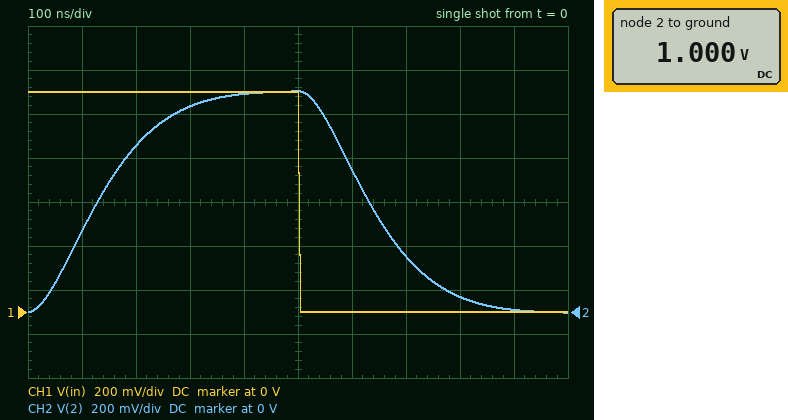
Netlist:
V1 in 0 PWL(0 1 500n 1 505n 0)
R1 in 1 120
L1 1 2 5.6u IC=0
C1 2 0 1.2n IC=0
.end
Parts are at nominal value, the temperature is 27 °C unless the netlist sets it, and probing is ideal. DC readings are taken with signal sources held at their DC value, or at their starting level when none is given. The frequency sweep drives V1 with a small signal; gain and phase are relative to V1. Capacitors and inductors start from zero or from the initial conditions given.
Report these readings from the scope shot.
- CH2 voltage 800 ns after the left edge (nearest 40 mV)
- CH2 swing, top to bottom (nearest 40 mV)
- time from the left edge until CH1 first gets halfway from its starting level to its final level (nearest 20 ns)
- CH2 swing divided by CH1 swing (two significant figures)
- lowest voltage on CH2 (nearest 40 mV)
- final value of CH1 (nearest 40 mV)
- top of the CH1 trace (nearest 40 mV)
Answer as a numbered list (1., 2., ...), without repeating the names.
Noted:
1. 80 mV
2. 1.00 V
3. 500 ns
4. 1.0
5. 0 V
6. 0 V
7. 1.00 V
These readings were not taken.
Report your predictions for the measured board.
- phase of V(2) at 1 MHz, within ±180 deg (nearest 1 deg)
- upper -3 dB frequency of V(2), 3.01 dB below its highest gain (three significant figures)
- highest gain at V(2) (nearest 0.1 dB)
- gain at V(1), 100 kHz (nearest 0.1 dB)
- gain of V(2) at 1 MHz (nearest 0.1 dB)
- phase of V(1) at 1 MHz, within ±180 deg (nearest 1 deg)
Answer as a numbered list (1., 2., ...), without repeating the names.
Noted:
1. -51 deg
2. 1.50 MHz
3. 0 dB
4. 0 dB
5. -1.3 dB
6. -51 deg
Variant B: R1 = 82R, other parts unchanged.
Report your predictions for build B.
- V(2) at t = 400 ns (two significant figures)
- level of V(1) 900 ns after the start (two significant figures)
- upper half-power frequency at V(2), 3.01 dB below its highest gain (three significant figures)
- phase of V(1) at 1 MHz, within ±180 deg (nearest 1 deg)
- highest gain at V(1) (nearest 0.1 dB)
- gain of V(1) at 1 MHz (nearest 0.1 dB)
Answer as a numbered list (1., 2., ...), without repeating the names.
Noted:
1. 1.1 V
2. -56 mV
3. 2.16 MHz
4. -40 deg
5. 0 dB
6. -2.3 dB
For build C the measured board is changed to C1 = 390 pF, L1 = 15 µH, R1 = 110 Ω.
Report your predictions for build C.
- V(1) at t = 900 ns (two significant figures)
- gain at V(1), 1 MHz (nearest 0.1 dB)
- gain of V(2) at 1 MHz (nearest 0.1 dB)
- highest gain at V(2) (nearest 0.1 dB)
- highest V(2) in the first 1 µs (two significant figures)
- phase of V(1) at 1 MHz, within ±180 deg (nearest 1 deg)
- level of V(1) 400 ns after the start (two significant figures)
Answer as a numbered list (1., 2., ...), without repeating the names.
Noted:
1. -110 mV
2. -0.5 dB
3. 1.8 dB
4. 5.4 dB
5. 1.4 V
6. -19 deg
7. 1.1 V
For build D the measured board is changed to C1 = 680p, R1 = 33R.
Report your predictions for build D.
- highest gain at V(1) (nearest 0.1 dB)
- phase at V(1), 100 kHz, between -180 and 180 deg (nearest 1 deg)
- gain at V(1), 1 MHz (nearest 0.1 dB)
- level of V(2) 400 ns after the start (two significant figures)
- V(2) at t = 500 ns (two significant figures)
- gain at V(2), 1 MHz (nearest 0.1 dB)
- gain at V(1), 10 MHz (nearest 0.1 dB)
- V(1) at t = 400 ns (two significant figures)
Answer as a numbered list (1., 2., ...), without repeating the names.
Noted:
1. 0 dB
2. -1 deg
3. -0.1 dB
4. 690 mV
5. 980 mV
6. 1.3 dB
7. 0 dB
8. 990 mV
